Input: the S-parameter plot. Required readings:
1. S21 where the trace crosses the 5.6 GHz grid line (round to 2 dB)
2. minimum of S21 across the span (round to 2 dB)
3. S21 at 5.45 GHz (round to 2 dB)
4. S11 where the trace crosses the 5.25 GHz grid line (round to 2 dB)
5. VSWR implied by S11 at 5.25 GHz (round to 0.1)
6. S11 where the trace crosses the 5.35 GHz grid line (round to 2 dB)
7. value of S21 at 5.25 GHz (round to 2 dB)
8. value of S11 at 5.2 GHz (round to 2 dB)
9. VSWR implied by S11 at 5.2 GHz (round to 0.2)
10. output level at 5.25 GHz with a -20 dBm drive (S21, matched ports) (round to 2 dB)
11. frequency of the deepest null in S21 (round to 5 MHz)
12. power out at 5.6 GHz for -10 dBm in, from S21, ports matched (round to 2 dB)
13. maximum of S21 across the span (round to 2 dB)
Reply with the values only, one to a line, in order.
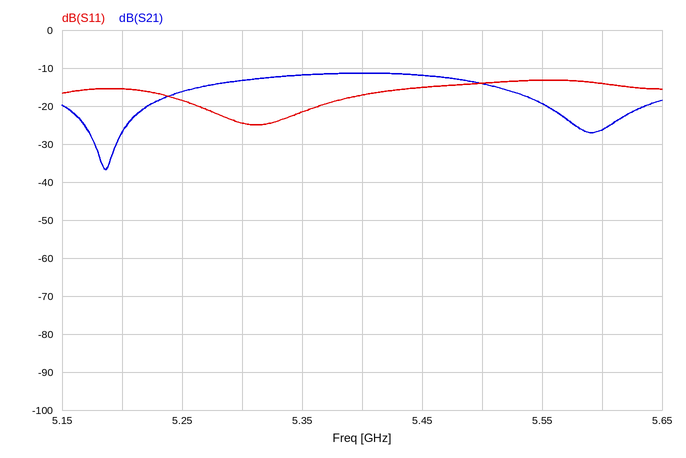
-26 dB
-36 dB
-12 dB
-18 dB
1.3
-22 dB
-16 dB
-16 dB
1.4
-36 dBm
5.185 GHz
-36 dBm
-12 dB
